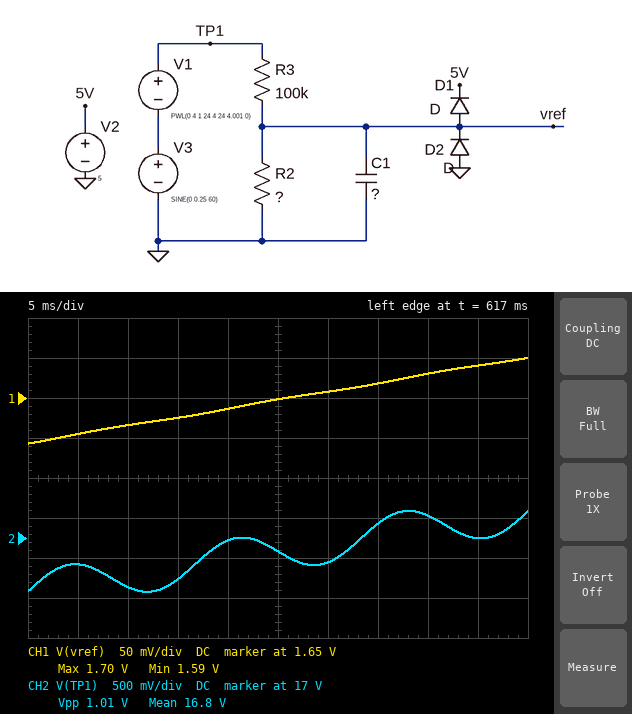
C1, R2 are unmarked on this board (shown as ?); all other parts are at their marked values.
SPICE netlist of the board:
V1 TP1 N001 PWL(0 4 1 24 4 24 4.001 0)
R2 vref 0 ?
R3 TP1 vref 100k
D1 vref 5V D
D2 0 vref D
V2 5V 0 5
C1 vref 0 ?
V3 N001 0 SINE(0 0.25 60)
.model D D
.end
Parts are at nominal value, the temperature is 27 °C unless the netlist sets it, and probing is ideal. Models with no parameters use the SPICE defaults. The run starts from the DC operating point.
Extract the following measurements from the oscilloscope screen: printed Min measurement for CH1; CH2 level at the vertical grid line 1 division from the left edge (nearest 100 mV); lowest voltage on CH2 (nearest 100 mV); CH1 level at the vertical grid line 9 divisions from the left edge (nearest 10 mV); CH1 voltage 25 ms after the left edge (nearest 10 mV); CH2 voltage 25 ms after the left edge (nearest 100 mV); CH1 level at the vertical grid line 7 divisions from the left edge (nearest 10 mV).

1.59 V
16.7 V
16.3 V
1.69 V
1.65 V
16.8 V
1.67 V
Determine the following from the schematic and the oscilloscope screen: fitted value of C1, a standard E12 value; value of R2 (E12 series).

6.8 µF
12 kΩ
